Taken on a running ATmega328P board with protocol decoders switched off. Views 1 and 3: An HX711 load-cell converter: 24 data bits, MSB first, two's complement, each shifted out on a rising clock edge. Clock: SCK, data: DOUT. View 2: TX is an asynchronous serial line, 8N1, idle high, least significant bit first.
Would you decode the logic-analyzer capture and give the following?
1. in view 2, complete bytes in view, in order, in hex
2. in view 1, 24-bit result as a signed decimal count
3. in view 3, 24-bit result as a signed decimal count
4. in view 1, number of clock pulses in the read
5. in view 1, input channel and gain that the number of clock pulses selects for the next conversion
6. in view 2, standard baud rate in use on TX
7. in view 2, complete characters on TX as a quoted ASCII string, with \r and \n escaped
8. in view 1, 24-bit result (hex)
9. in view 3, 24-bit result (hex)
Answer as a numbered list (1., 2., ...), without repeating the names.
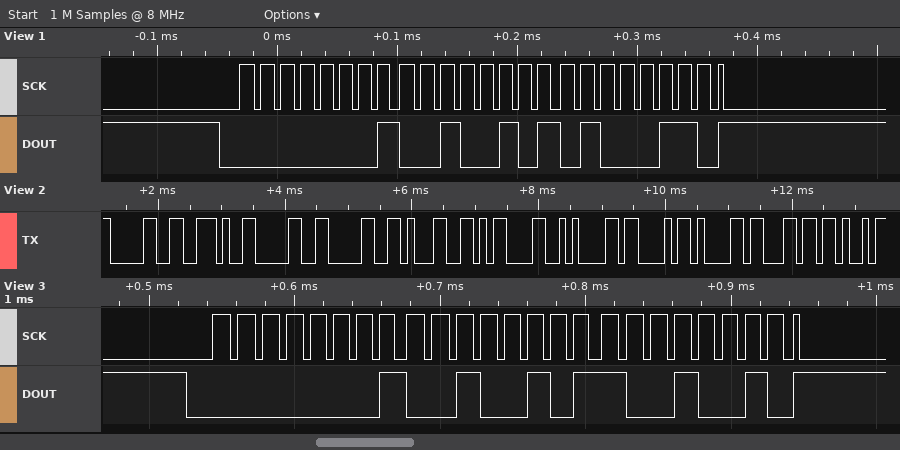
1. 30 2E 30 30 31 0D 0A 43 61 6C
2. 75078
3. 75154
4. 25
5. channel A, gain 128
6. 9600 baud
7. "0.001\r\nCal"
8. 0x012546
9. 0x012592
